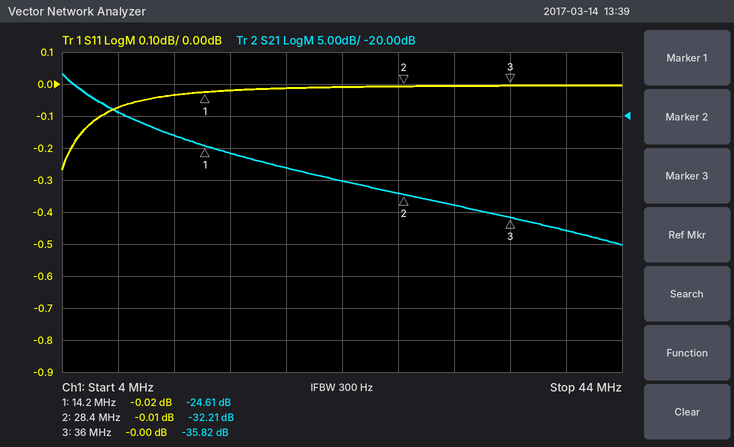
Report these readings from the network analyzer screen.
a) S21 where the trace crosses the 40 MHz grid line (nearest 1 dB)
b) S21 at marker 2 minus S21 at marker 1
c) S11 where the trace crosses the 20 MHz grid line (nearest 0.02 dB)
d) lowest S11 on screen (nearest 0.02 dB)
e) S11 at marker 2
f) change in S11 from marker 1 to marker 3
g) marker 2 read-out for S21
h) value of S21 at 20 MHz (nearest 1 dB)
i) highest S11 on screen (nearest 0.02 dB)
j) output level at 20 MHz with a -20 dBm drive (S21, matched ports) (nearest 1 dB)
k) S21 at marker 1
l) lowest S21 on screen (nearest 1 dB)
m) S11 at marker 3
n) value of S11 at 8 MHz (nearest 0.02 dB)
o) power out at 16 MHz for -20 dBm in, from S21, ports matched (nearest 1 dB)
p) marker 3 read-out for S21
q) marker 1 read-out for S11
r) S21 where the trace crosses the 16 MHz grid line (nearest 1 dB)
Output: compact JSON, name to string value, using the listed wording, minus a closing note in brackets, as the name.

{"S21 where the trace crosses the 40 MHz grid line": "-38 dB", "S21 at marker 2 minus S21 at marker 1": "-7.60 dB", "S11 where the trace crosses the 20 MHz grid line": "-0.02 dB", "lowest S11 on screen": "-0.26 dB", "S11 at marker 2": "-0.01 dB", "change in S11 from marker 1 to marker 3": "0.02 dB", "marker 2 read-out for S21": "-32.21 dB", "value of S21 at 20 MHz": "-28 dB", "highest S11 on screen": "0.00 dB", "output level at 20 MHz with a -20 dBm drive (S21, matched ports)": "-48 dBm", "S21 at marker 1": "-24.61 dB", "lowest S21 on screen": "-40 dB", "S11 at marker 3": "-0.00 dB", "value of S11 at 8 MHz": "-0.08 dB", "power out at 16 MHz for -20 dBm in, from S21, ports matched": "-46 dBm", "marker 3 read-out for S21": "-35.82 dB", "marker 1 read-out for S11": "-0.02 dB", "S21 where the trace crosses the 16 MHz grid line": "-26 dB"}
